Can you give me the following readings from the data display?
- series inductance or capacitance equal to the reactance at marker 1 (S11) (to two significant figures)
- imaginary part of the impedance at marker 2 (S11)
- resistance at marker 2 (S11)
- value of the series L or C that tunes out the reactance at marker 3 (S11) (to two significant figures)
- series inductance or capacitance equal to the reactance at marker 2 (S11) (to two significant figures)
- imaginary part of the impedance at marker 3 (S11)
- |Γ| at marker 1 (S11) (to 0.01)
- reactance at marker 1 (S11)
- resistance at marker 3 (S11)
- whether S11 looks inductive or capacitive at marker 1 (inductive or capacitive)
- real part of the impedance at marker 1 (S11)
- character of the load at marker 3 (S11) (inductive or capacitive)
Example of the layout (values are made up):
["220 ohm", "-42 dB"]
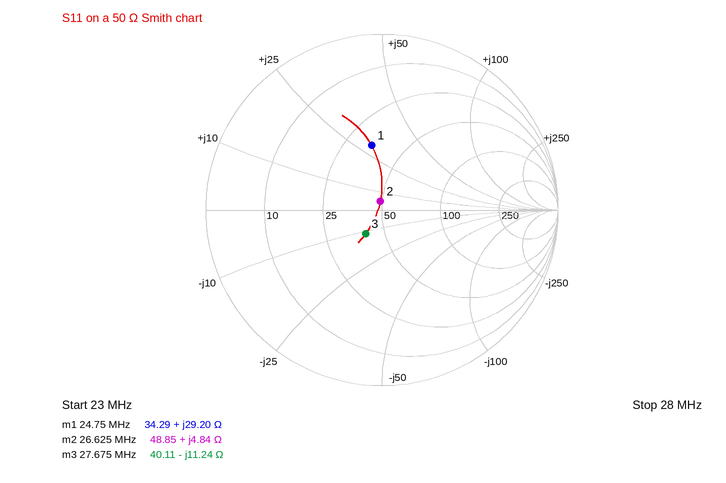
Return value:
["190 nH", "+4.84 Ω", "48.85 Ω", "65 nH", "29 nH", "-11.24 Ω", "0.37", "+29.20 Ω", "40.11 Ω", "inductive", "34.29 Ω", "capacitive"]
